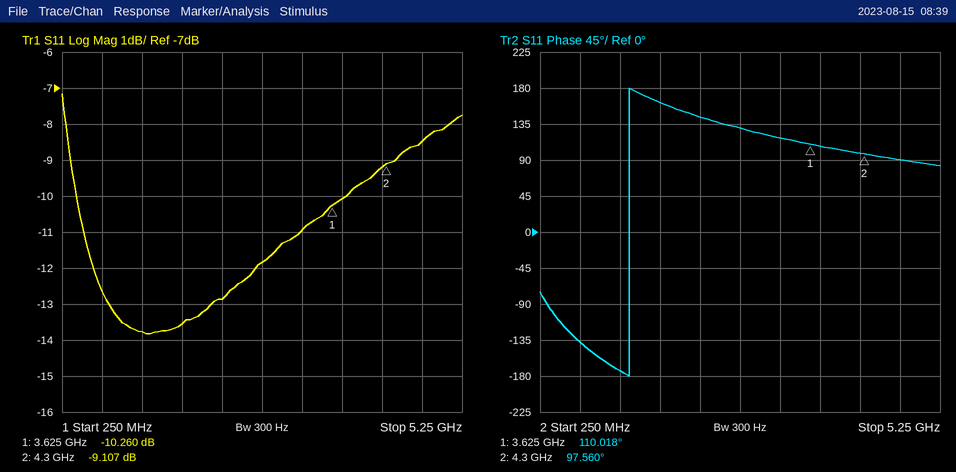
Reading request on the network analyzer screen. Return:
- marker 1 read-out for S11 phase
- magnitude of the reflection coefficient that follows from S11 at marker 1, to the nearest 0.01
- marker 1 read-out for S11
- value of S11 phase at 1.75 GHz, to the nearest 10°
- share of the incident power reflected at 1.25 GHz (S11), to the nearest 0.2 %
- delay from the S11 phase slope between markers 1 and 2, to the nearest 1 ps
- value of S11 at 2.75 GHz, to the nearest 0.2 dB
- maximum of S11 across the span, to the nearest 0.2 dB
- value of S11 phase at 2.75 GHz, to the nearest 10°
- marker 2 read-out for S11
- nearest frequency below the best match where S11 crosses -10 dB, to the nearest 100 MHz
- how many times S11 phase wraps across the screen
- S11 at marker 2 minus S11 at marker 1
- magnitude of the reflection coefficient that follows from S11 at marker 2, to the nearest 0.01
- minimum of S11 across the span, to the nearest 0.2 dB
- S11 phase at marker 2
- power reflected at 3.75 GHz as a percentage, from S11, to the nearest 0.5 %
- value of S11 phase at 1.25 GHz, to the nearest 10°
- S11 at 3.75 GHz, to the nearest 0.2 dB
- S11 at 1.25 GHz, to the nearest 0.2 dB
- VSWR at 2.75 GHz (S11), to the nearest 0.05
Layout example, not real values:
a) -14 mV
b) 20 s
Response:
a) 110.018°
b) 0.31
c) -10.260 dB
d) 160°
e) 4.2 %
f) 51 ps
g) -11.8 dB
h) -7.2 dB
i) 130°
j) -9.107 dB
k) 400 MHz
l) 1
m) 1.153 dB
n) 0.35
o) -13.8 dB
p) 97.560°
q) 10.0 %
r) -170°
s) -10.0 dB
t) -13.8 dB
u) 1.70
